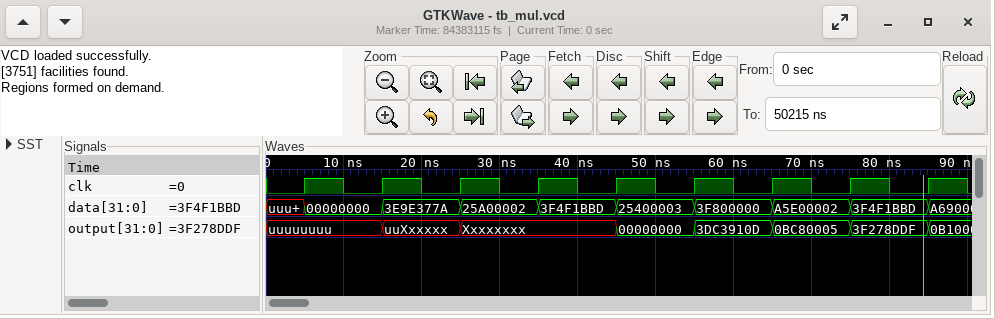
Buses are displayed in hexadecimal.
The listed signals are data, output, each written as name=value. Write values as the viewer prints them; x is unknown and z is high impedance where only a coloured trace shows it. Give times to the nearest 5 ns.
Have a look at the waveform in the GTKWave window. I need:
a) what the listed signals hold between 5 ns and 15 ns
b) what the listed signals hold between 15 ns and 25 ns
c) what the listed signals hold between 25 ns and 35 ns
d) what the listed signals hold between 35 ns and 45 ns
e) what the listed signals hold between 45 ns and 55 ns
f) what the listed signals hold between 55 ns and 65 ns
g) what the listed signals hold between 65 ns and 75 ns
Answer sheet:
data=00000000, output=uuuuuuuu
data=3E9E377A, output=uuXxxxxx
data=25A00002, output=Xxxxxxxx
data=3F4F1BBD, output=Xxxxxxxx
data=25400003, output=00000000
data=3F800000, output=3DC3910D
data=A5E00002, output=0BC80005
